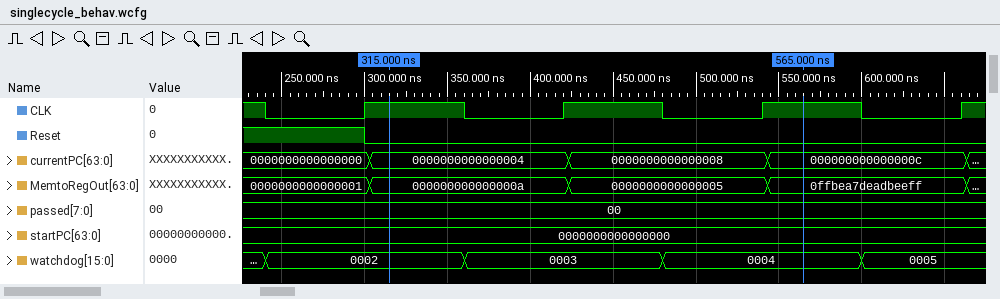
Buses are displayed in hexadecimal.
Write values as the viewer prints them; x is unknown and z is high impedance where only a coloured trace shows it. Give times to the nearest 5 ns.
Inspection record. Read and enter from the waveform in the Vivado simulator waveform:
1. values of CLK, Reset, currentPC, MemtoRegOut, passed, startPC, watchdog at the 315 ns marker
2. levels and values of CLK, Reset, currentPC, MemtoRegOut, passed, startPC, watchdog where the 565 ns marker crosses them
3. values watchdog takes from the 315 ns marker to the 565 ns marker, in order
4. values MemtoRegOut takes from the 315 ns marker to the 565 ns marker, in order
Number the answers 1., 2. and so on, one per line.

1. CLK=1, Reset=0, currentPC=0000000000000004, MemtoRegOut=000000000000000a, passed=00, startPC=0000000000000000, watchdog=0002
2. CLK=1, Reset=0, currentPC=000000000000000c, MemtoRegOut=0ffbea7deadbeeff, passed=00, startPC=0000000000000000, watchdog=0004
3. 0002, 0003, 0004
4. 000000000000000a, 0000000000000005, 0ffbea7deadbeeff
